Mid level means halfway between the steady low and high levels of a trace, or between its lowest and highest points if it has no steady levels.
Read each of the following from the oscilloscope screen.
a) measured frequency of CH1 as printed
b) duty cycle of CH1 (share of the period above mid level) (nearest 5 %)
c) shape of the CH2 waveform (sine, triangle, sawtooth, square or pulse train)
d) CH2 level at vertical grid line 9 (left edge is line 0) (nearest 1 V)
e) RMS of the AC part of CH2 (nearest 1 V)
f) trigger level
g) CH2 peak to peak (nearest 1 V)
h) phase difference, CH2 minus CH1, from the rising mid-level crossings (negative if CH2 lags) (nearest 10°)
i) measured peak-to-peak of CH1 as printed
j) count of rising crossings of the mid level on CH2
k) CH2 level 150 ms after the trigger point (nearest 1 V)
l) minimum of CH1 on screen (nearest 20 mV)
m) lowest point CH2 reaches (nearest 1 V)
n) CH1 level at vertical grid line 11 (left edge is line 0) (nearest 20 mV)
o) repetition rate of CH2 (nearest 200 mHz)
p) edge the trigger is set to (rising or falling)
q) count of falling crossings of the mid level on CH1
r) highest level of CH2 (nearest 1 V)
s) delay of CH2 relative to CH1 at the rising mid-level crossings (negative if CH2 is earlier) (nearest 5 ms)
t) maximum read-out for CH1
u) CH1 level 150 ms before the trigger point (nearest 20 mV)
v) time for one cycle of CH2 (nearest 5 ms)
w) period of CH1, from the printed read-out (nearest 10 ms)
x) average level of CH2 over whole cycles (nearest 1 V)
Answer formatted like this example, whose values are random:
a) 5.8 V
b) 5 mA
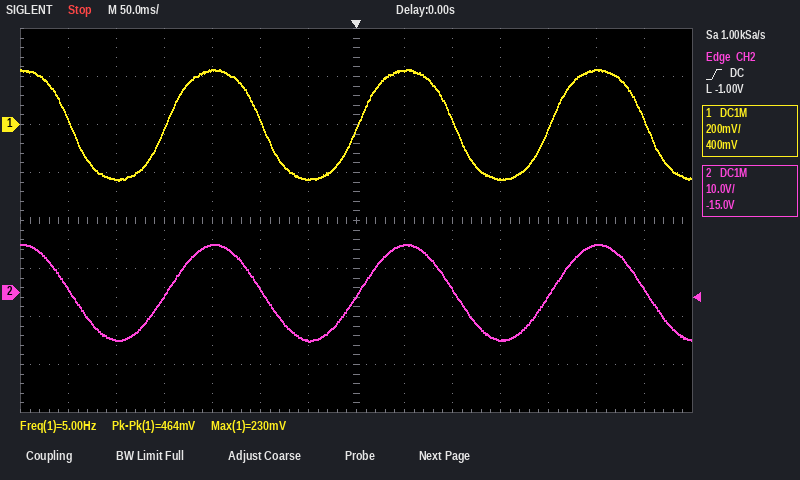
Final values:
a) 5.00 Hz
b) 50 %
c) sine
d) 1 V
e) 7 V
f) -1.00 V
g) 20 V
h) 0°
i) 464 mV
j) 3
k) -10 V
l) -240 mV
m) -10 V
n) -20 mV
o) 5.0 Hz
p) rising
q) 4
r) 10 V
s) 0 ms
t) 230 mV
u) 220 mV
v) 200 ms
w) 200 ms
x) 0 V
